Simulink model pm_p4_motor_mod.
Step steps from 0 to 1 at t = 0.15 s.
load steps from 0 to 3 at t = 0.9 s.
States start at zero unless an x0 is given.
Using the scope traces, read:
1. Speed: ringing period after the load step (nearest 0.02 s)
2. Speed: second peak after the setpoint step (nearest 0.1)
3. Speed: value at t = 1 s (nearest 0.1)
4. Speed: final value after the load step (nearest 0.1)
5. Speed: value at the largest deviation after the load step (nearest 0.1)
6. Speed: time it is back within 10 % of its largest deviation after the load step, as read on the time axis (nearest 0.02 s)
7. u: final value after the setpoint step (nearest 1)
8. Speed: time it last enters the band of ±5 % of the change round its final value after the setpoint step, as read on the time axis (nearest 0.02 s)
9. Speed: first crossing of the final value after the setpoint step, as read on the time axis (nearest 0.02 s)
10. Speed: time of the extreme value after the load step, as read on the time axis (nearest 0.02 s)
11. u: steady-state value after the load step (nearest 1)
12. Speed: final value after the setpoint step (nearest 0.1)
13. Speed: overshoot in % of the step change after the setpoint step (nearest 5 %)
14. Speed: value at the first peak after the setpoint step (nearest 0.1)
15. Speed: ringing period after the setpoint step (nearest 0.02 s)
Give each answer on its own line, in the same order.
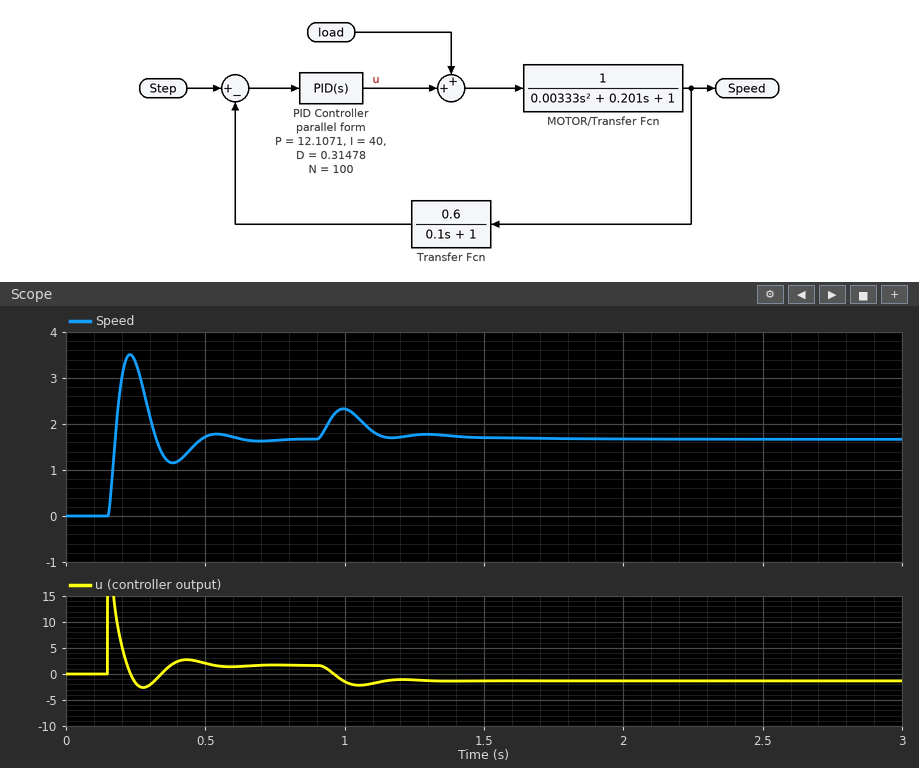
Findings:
0.30 s
1.8
2.3
1.7
2.3
1.40 s
2
0.58 s
0.18 s
1.00 s
-1
1.7
110 %
3.5
0.32 s
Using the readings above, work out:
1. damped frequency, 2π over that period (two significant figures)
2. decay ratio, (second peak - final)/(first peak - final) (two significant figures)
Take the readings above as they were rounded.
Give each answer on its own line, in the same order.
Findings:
20 rad/s
0.056
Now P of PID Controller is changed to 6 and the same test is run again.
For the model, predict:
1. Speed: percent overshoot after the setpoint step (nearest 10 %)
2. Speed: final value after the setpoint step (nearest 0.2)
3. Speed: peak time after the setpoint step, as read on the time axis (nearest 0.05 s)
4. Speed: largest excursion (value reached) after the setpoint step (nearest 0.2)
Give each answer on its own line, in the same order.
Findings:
50 %
1.6
0.25 s
2.6
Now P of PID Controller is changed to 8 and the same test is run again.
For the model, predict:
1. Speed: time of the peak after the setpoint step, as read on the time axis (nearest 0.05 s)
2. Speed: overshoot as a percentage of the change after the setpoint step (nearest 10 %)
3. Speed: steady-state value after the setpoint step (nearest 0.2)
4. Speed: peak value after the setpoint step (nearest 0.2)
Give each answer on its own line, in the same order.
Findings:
0.25 s
70 %
1.6
2.8
